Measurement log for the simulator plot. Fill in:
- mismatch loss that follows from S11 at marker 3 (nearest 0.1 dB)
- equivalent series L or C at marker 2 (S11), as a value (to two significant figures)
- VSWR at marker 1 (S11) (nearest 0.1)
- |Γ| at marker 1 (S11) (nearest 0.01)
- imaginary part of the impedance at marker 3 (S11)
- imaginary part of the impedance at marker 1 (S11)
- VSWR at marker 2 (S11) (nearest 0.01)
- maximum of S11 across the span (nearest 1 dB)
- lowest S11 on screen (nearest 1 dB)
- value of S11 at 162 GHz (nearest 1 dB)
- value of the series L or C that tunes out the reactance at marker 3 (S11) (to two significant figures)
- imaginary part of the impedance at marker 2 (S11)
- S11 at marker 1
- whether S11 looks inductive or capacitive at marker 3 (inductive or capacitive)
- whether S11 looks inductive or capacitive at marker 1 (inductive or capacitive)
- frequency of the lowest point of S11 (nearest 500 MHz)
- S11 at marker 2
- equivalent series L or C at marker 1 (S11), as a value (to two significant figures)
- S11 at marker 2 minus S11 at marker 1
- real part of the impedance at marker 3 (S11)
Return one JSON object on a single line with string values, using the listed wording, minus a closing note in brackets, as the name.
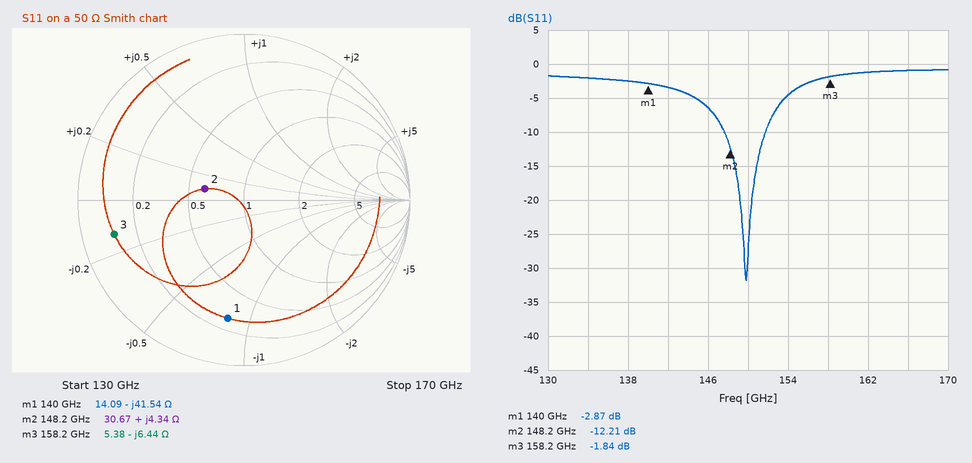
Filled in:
{"mismatch loss that follows from S11 at marker 3": "4.6 dB", "equivalent series L or C at marker 2 (S11), as a value": "4.7 pH", "VSWR at marker 1 (S11)": "6.1", "|Γ| at marker 1 (S11)": "0.72", "imaginary part of the impedance at marker 3": "-6.44 Ω", "imaginary part of the impedance at marker 1": "-41.54 Ω", "VSWR at marker 2 (S11)": "1.65", "maximum of S11 across the span": "-1 dB", "lowest S11 on screen": "-32 dB", "value of S11 at 162 GHz": "-1 dB", "value of the series L or C that tunes out the reactance at marker 3 (S11)": "6.5 pH", "imaginary part of the impedance at marker 2": "+4.34 Ω", "S11 at marker 1": "-2.87 dB", "whether S11 looks inductive or capacitive at marker 3": "capacitive", "whether S11 looks inductive or capacitive at marker 1": "capacitive", "frequency of the lowest point of S11": "150.0 GHz", "S11 at marker 2": "-12.21 dB", "equivalent series L or C at marker 1 (S11), as a value": "27 fF", "S11 at marker 2 minus S11 at marker 1": "-9.34 dB", "real part of the impedance at marker 3": "5.38 Ω"}
